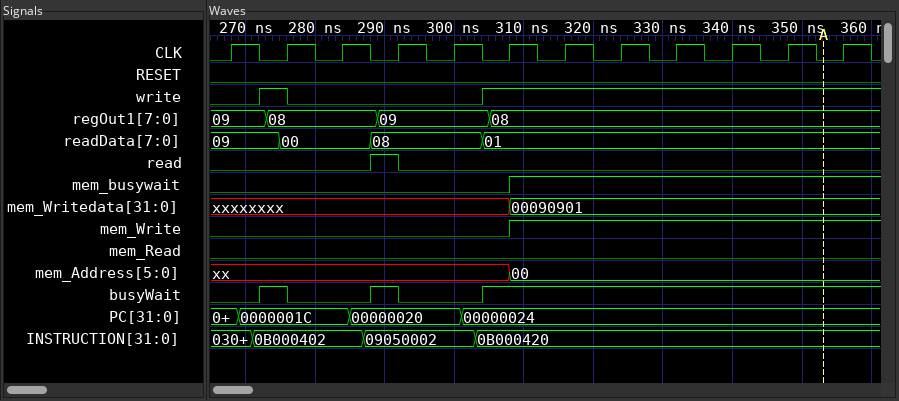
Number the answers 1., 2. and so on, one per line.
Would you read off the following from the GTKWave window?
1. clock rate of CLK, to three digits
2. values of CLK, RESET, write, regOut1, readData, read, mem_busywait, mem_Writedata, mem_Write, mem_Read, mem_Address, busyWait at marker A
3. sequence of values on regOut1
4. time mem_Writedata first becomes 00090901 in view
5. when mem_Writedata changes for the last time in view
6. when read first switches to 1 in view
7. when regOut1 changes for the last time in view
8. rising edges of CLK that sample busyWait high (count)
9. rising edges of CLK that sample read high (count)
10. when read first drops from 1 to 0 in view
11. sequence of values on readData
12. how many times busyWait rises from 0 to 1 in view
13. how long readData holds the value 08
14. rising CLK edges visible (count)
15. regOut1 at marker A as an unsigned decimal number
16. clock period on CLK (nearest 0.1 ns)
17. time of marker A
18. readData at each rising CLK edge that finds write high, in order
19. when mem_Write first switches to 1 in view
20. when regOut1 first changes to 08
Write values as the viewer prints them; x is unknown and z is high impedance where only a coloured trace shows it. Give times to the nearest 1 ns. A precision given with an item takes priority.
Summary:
1. 125 MHz
2. CLK=0, RESET=0, write=1, regOut1=08, readData=01, read=0, mem_busywait=1, mem_Writedata=00090901, mem_Write=1, mem_Read=0, mem_Address=00, busyWait=1
3. 09, 08, 09, 08
4. 308 ns
5. 308 ns
6. 288 ns
7. 305 ns
8. 9
9. 1
10. 292 ns
11. 09, 00, 08, 01
12. 3
13. 16 ns
14. 12
15. 8
16. 8 ns
17. 353 ns
18. 00, 01, 01, 01, 01, 01, 01, 01
19. 308 ns
20. 273 ns
